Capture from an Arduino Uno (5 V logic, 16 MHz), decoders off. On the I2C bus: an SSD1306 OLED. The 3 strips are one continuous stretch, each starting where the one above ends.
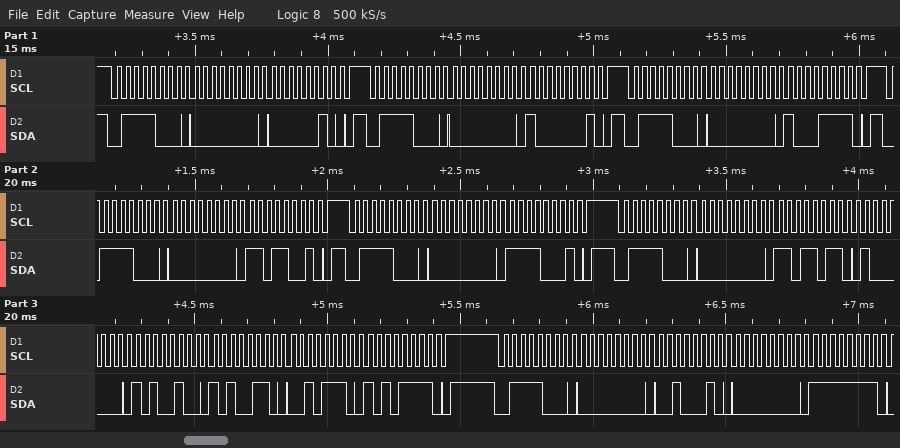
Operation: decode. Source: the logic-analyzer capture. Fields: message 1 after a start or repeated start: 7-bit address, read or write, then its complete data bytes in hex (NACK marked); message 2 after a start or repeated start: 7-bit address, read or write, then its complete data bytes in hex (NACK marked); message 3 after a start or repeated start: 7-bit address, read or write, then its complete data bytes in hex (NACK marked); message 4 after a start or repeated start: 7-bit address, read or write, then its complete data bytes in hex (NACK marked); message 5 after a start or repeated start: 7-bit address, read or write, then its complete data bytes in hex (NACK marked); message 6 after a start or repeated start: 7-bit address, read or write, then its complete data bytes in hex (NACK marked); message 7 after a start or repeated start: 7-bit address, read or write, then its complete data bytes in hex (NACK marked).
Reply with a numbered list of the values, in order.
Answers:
1. 0x3C write: 00 02
2. 0x3C write: 00 81
3. 0x3C write: 00 8F
4. 0x3C write: 00 D9
5. 0x3C write: 00 F1
6. 0x3C write: 00 DB 40 A4 A6 2E AF
7. 0x3C write: 00 22 00 FF
